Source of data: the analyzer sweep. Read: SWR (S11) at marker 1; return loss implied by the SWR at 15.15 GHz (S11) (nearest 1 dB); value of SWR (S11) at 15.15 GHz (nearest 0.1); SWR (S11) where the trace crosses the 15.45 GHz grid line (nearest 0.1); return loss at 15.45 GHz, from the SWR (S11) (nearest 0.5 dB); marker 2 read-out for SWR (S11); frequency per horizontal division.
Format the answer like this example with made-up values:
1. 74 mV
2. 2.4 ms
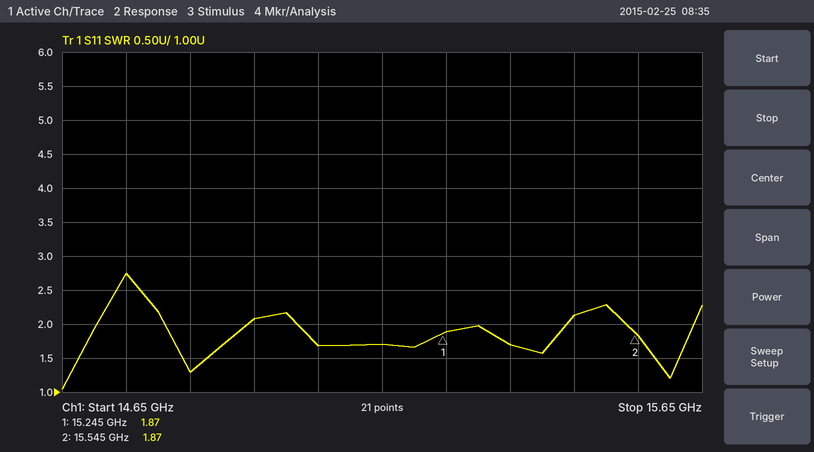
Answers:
1. 1.87
2. 12 dB
3. 1.7
4. 2.1
5. 9.0 dB
6. 1.87
7. 100 MHz
